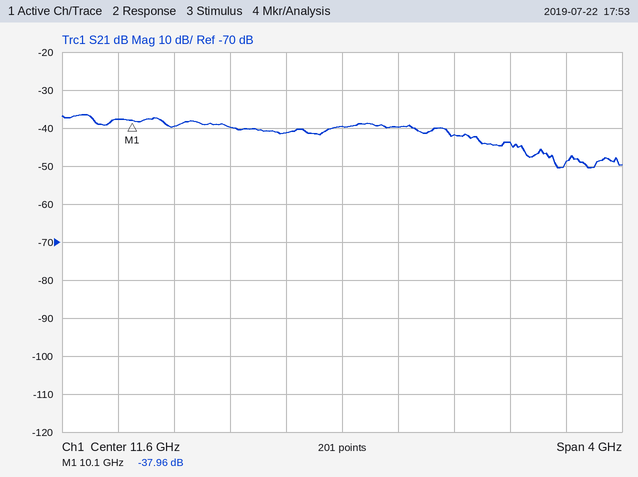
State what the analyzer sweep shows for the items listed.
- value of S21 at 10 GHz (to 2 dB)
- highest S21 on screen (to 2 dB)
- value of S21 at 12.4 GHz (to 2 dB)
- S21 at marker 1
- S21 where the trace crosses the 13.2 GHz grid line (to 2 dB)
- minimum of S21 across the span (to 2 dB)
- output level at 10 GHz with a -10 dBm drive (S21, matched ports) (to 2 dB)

-38 dB
-36 dB
-42 dB
-37.96 dB
-48 dB
-50 dB
-48 dBm
